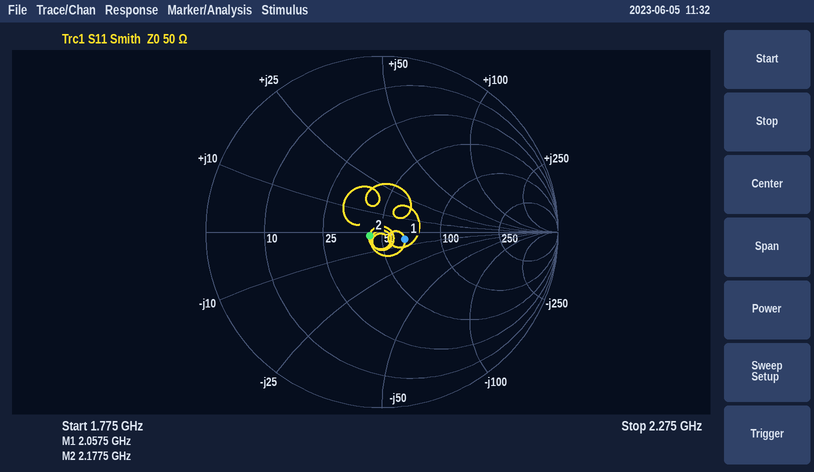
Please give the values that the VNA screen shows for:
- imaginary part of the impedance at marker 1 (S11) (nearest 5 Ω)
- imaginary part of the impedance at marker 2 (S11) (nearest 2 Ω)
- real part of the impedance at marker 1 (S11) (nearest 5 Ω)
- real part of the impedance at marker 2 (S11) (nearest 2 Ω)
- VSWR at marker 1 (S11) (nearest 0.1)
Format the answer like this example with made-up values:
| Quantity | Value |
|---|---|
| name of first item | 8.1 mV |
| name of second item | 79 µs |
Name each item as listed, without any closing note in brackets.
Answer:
| Quantity | Value |
|---|---|
| imaginary part of the impedance at marker 1 (S11) | -5 Ω |
| imaginary part of the impedance at marker 2 (S11) | -2 Ω |
| real part of the impedance at marker 1 (S11) | 65 Ω |
| real part of the impedance at marker 2 (S11) | 44 Ω |
| VSWR at marker 1 (S11) | 1.3 |
